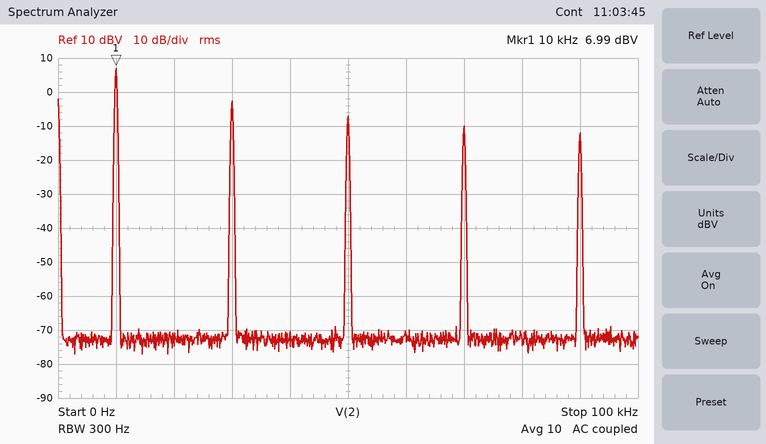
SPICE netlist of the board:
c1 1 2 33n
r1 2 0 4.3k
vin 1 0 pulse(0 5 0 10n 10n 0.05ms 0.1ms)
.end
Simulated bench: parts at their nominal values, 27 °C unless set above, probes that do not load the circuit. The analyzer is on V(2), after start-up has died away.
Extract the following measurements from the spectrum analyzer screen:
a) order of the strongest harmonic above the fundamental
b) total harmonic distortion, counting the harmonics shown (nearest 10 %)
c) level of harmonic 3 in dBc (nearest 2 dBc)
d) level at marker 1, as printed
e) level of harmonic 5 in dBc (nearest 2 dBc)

3
40 %
-10 dBc
6.99 dBV
-14 dBc
